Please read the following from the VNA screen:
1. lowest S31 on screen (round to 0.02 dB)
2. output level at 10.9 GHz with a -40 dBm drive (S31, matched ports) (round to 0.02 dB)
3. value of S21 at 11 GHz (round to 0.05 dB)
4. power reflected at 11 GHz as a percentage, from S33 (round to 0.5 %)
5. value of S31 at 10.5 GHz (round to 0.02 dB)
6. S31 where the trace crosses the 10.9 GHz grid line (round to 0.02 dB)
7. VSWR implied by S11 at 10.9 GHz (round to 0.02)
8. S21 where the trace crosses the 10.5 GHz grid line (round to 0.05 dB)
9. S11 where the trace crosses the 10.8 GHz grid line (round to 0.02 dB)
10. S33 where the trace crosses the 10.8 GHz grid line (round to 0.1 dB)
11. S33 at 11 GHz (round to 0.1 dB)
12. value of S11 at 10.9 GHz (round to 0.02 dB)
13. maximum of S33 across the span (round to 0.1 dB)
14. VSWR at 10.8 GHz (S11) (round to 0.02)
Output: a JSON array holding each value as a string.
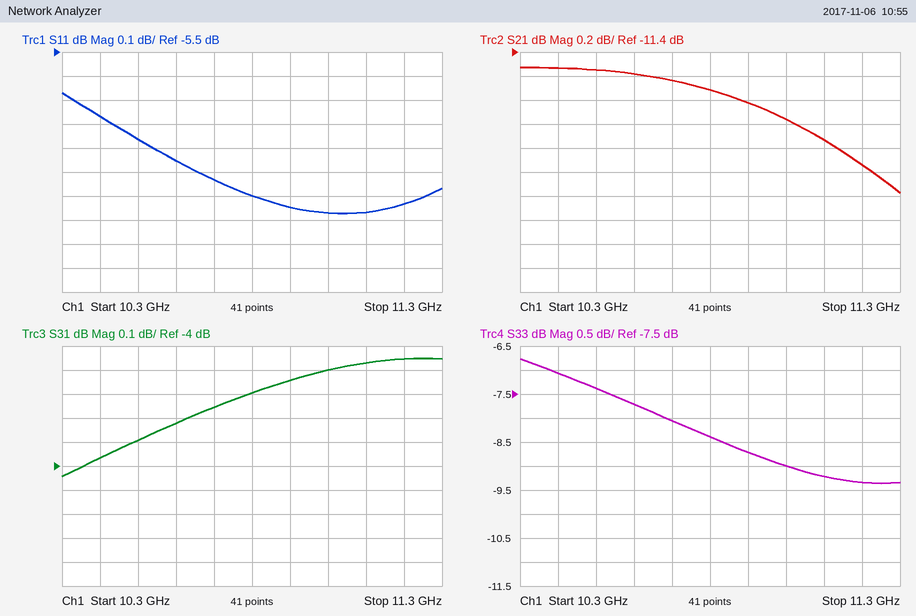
["-4.04 dB", "-43.64 dBm", "-11.95 dB", "12.5 %", "-3.90 dB", "-3.64 dB", "2.94", "-11.55 dB", "-6.10 dB", "-8.4 dB", "-9.0 dB", "-6.14 dB", "-6.8 dB", "2.96"]
